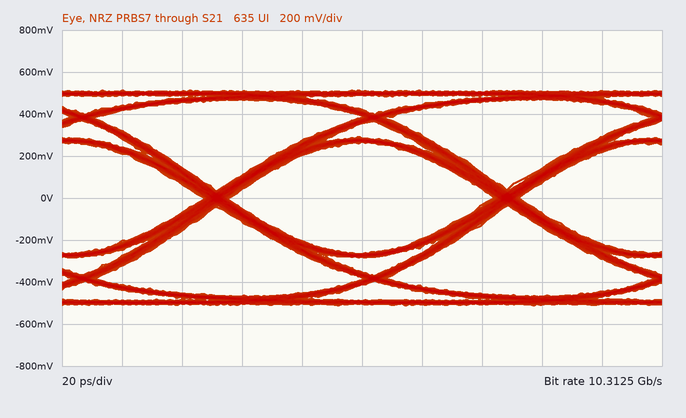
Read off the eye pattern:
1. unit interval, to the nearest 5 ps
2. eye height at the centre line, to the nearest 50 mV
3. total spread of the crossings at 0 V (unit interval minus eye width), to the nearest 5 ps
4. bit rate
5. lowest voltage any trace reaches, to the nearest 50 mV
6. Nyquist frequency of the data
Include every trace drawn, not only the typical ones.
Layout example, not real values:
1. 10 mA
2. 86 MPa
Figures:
1. 95 ps
2. 550 mV
3. 10 ps
4. 10.3125 Gb/s
5. -500 mV
6. 5.15625 GHz
